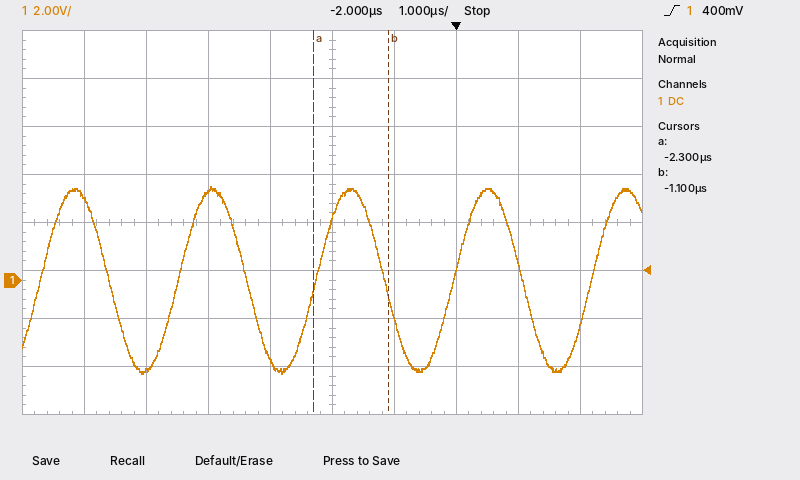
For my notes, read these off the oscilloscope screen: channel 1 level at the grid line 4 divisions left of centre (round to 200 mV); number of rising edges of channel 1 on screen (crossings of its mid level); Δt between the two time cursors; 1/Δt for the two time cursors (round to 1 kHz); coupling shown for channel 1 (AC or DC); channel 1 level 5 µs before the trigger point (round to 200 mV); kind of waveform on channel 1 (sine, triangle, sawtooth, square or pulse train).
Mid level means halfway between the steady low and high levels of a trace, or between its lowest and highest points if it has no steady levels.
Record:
3.4 V
5
1.2 µs
833 kHz
DC
-3.8 V
sine
